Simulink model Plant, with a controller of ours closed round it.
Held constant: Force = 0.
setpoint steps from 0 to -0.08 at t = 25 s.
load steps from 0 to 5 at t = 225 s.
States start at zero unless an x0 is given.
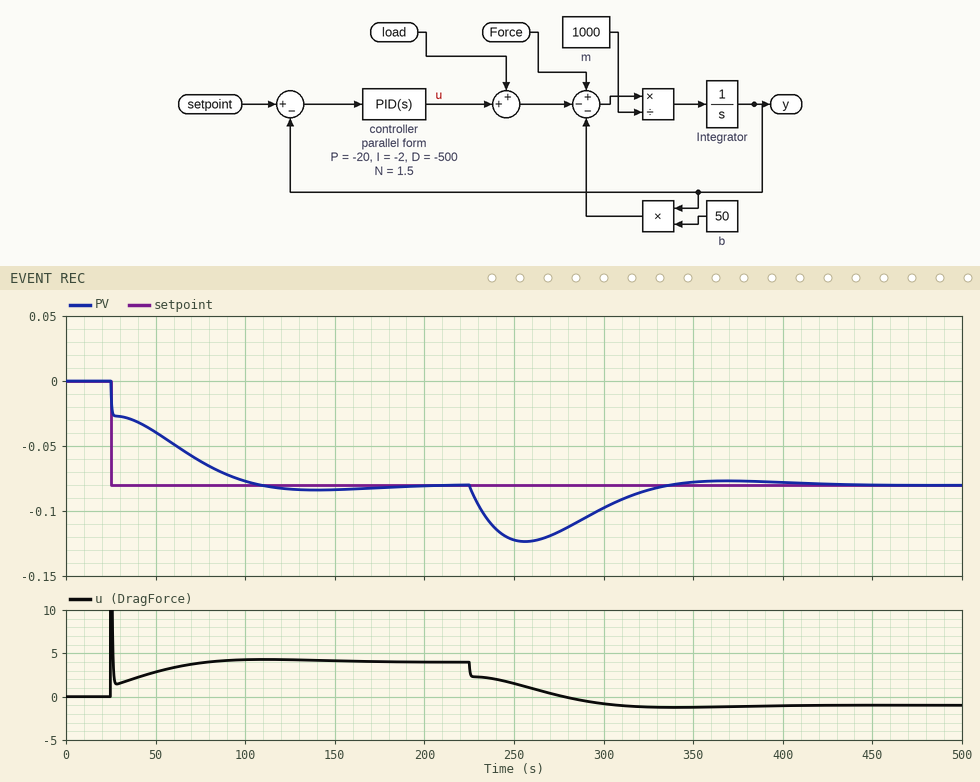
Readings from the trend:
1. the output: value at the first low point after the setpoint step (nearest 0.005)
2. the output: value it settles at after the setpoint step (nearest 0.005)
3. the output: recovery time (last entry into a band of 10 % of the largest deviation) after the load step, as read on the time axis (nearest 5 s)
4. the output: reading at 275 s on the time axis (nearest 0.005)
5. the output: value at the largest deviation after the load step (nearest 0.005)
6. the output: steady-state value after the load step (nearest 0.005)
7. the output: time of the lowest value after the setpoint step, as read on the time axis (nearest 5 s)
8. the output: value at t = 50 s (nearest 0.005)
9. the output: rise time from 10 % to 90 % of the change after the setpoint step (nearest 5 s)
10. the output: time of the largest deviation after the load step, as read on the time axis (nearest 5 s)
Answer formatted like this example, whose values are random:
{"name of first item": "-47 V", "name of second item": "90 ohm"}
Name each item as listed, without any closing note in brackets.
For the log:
{"the output: value at the first low point after the setpoint step": "-0.085", "the output: value it settles at after the setpoint step": "-0.080", "the output: recovery time (last entry into a band of 10 % of the largest deviation) after the load step, as read on the time axis": "325 s", "the output: reading at 275 s on the time axis": "-0.115", "the output: value at the largest deviation after the load step": "-0.125", "the output: steady-state value after the load step": "-0.080", "the output: time of the lowest value after the setpoint step, as read on the time axis": "140 s", "the output: value at t = 50 s": "-0.040", "the output: rise time from 10 % to 90 % of the change after the setpoint step": "65 s", "the output: time of the largest deviation after the load step, as read on the time axis": "255 s"}
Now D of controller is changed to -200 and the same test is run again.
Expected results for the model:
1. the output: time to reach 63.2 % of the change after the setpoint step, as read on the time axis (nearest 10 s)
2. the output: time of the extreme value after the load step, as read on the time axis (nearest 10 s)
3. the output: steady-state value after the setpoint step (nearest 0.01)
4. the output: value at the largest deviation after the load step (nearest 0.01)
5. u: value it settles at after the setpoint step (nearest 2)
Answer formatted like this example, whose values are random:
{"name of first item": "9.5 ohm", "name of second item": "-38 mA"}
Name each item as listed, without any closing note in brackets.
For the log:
{"the output: time to reach 63.2 % of the change after the setpoint step, as read on the time axis": "60 s", "the output: time of the extreme value after the load step, as read on the time axis": "250 s", "the output: steady-state value after the setpoint step": "-0.08", "the output: value at the largest deviation after the load step": "-0.13", "u: value it settles at after the setpoint step": "4"}
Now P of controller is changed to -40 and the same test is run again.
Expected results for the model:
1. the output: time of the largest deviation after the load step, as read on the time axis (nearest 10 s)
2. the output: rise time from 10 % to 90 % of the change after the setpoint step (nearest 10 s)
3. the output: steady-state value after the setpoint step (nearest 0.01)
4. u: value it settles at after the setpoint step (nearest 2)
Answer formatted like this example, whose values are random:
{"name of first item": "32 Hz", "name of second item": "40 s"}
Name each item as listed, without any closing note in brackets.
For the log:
{"the output: time of the largest deviation after the load step, as read on the time axis": "250 s", "the output: rise time from 10 % to 90 % of the change after the setpoint step": "70 s", "the output: steady-state value after the setpoint step": "-0.08", "u: value it settles at after the setpoint step": "4"}
